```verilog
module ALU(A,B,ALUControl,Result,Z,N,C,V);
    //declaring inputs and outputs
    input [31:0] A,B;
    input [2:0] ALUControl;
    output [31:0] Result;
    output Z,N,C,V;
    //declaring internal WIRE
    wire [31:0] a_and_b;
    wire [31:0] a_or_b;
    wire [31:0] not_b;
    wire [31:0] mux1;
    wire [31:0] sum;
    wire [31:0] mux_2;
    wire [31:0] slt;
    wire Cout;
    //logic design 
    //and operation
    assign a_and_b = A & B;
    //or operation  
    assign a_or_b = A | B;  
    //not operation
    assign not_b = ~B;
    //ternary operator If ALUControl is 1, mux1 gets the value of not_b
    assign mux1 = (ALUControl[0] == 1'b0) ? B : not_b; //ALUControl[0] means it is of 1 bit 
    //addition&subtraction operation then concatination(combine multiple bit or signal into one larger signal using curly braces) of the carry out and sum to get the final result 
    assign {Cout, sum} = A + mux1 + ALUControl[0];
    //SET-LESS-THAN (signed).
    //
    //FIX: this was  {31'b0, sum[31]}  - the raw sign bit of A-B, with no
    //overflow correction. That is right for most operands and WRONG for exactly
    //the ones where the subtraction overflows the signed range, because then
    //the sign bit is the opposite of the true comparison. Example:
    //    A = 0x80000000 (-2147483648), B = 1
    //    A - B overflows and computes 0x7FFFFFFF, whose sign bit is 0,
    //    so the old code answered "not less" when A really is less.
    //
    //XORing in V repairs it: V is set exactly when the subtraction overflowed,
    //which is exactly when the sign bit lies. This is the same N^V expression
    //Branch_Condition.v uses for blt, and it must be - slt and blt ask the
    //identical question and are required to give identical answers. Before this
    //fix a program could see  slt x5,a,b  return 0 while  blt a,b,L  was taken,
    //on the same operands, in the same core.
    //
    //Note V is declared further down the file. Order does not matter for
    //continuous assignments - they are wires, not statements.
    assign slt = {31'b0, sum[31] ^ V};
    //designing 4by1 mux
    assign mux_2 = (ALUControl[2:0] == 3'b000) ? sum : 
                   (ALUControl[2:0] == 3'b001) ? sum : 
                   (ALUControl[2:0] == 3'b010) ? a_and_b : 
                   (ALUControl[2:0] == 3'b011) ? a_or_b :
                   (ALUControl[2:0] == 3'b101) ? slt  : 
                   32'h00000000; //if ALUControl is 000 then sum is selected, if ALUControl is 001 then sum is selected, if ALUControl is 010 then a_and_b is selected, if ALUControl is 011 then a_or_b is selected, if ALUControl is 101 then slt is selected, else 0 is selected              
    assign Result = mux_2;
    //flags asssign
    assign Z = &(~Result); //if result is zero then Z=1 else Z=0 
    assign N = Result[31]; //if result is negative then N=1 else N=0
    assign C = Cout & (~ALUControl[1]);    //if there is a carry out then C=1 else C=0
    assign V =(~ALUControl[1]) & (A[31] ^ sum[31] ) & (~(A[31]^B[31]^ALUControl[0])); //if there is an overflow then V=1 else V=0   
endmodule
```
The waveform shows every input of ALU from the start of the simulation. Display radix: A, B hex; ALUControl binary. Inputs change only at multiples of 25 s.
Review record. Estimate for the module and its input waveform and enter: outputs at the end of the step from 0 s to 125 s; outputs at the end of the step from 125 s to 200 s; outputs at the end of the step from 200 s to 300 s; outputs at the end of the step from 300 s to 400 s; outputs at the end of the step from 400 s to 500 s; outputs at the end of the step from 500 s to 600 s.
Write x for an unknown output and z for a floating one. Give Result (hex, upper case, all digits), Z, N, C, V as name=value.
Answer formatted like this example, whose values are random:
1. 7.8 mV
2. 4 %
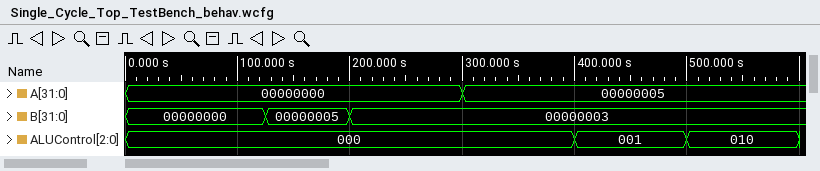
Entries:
1. Result=00000000, Z=1, N=0, C=0, V=0
2. Result=00000005, Z=0, N=0, C=0, V=0
3. Result=00000003, Z=0, N=0, C=0, V=0
4. Result=00000008, Z=0, N=0, C=0, V=0
5. Result=00000002, Z=0, N=0, C=1, V=0
6. Result=00000001, Z=0, N=0, C=0, V=0
